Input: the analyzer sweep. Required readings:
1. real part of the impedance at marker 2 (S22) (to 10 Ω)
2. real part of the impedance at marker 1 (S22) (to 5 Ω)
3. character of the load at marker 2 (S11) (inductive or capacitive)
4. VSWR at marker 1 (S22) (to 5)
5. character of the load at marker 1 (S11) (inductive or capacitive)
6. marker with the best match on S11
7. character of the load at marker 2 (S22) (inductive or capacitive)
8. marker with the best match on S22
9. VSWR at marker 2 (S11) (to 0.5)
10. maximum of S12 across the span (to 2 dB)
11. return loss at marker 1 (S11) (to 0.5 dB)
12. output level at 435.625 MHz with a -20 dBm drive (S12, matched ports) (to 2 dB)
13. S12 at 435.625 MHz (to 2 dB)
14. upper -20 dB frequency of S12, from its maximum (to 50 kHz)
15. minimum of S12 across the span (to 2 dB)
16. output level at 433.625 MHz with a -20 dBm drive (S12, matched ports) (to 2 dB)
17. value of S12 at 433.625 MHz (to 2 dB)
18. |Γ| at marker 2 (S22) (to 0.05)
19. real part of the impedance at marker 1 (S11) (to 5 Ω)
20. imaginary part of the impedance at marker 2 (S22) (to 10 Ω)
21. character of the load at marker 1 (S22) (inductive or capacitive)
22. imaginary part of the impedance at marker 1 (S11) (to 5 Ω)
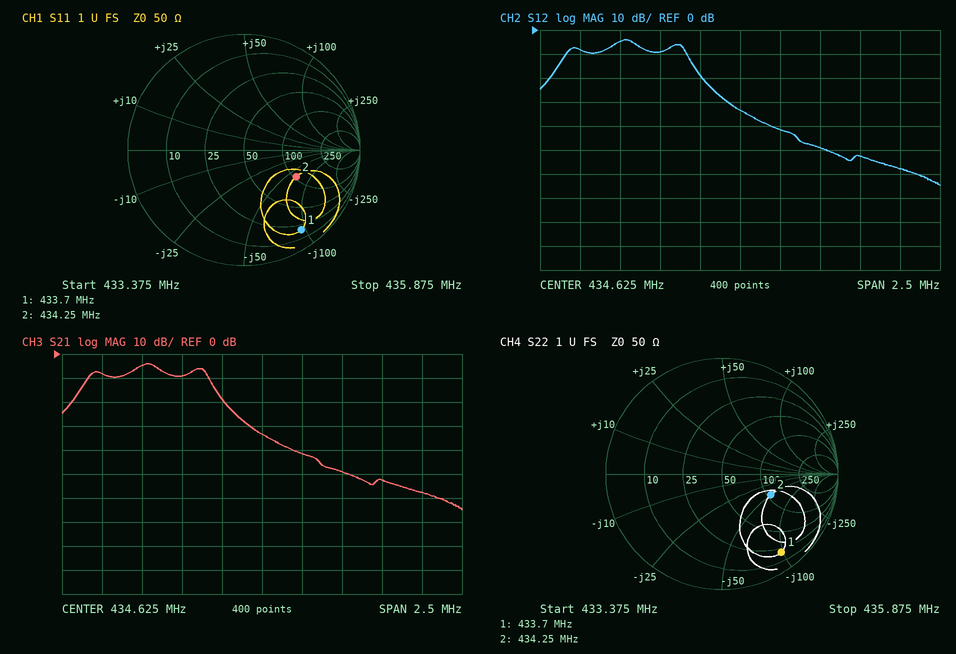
110 Ω
20 Ω
capacitive
10
capacitive
marker 2
capacitive
marker 2
3.0
-4 dB
1.5 dB
-78 dBm
-58 dB
434.45 MHz
-64 dB
-28 dBm
-8 dB
0.45
20 Ω
-50 Ω
capacitive
-95 Ω
